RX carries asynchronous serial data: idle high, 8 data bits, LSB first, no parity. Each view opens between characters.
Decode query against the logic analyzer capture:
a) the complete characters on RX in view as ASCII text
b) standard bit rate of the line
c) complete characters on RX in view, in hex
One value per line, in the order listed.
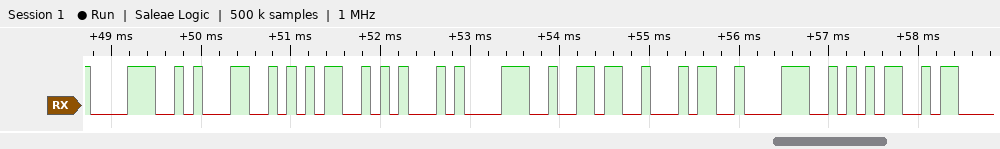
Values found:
"815E86485"
9600 baud
38, 31, 35, 45, 38, 36, 34, 38, 35
